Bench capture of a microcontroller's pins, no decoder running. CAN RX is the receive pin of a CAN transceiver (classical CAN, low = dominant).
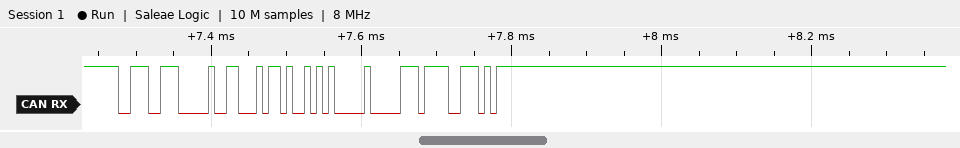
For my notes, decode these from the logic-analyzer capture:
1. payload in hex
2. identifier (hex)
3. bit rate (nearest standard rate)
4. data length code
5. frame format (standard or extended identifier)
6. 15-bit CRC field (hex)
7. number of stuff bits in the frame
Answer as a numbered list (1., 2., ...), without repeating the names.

1. 16 95 00
2. 0x39C
3. 125 kbit/s
4. 3
5. standard
6. 0x1BCE
7. 3
